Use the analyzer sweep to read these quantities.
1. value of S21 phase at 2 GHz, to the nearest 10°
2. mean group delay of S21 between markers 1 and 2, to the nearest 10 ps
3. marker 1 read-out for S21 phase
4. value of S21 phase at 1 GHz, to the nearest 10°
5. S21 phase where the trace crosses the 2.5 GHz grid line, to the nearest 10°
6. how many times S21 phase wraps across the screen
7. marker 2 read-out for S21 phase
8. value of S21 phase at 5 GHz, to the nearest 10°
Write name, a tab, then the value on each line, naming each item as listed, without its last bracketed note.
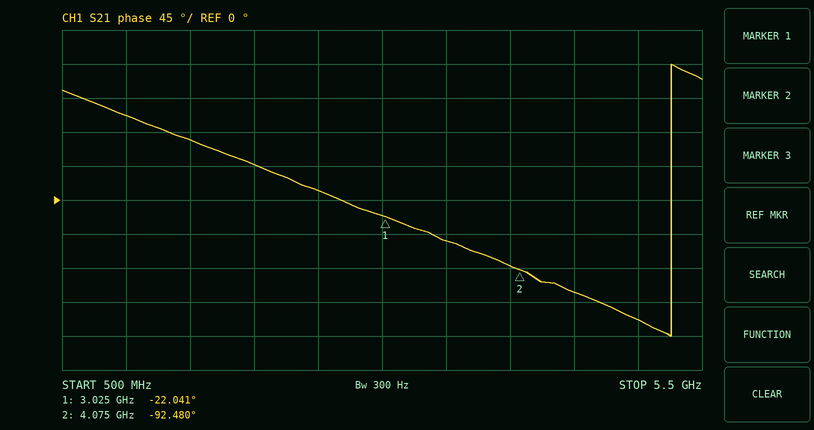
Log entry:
value of S21 phase at 2 GHz, to the nearest 10°	50°
mean group delay of S21 between markers 1 and 2, to the nearest 10 ps	190 ps
marker 1 read-out for S21 phase	-22.041°
value of S21 phase at 1 GHz, to the nearest 10°	110°
S21 phase where the trace crosses the 2.5 GHz grid line, to the nearest 10°	10°
how many times S21 phase wraps across the screen	1
marker 2 read-out for S21 phase	-92.480°
value of S21 phase at 5 GHz, to the nearest 10°	-160°
